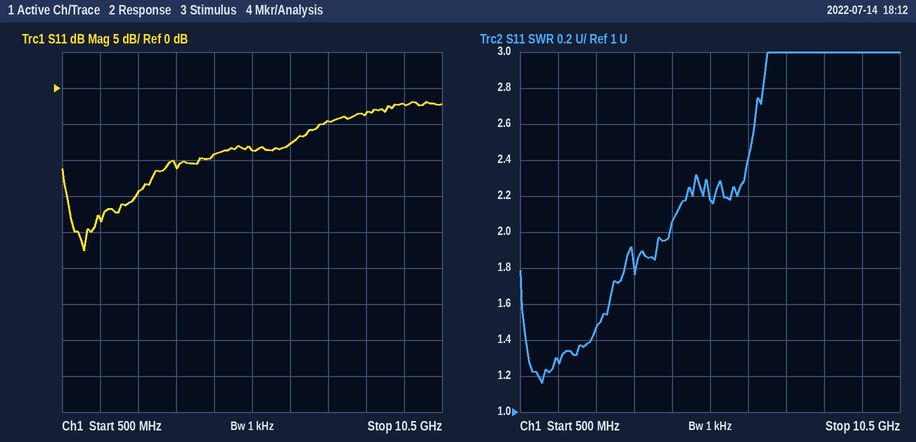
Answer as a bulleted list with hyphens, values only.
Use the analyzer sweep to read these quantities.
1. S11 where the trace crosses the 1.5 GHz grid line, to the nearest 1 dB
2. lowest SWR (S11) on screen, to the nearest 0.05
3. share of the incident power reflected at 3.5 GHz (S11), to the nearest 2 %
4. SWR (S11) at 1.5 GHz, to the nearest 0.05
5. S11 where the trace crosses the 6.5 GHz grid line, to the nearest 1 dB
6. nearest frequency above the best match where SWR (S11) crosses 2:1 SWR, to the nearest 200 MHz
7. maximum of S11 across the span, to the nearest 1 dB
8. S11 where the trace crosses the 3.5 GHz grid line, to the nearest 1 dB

- -18 dB
- 1.15
- 8 %
- 1.30
- -8 dB
- 4.4 GHz
- -2 dB
- -11 dB
